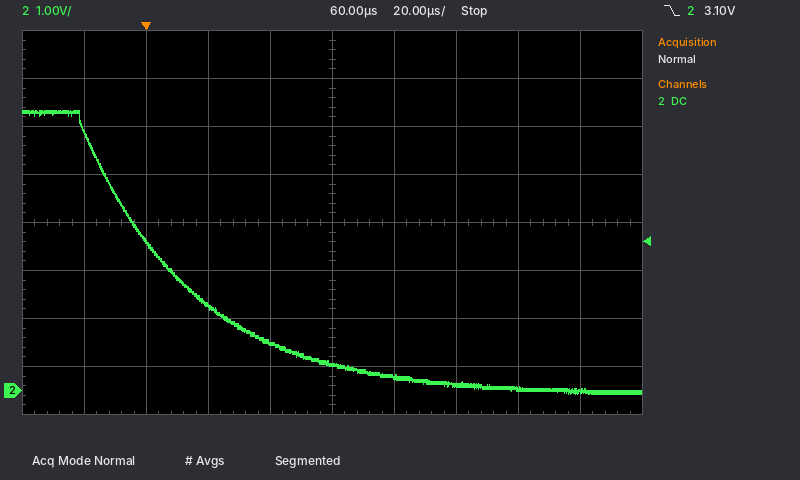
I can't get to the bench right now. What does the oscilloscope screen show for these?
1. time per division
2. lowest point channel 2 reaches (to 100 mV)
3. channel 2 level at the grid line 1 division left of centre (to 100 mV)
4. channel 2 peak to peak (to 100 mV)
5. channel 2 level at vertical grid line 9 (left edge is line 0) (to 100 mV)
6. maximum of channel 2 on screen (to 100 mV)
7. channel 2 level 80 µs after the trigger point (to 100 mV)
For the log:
20 µs
-100 mV
1.0 V
5.9 V
0.0 V
5.8 V
300 mV
